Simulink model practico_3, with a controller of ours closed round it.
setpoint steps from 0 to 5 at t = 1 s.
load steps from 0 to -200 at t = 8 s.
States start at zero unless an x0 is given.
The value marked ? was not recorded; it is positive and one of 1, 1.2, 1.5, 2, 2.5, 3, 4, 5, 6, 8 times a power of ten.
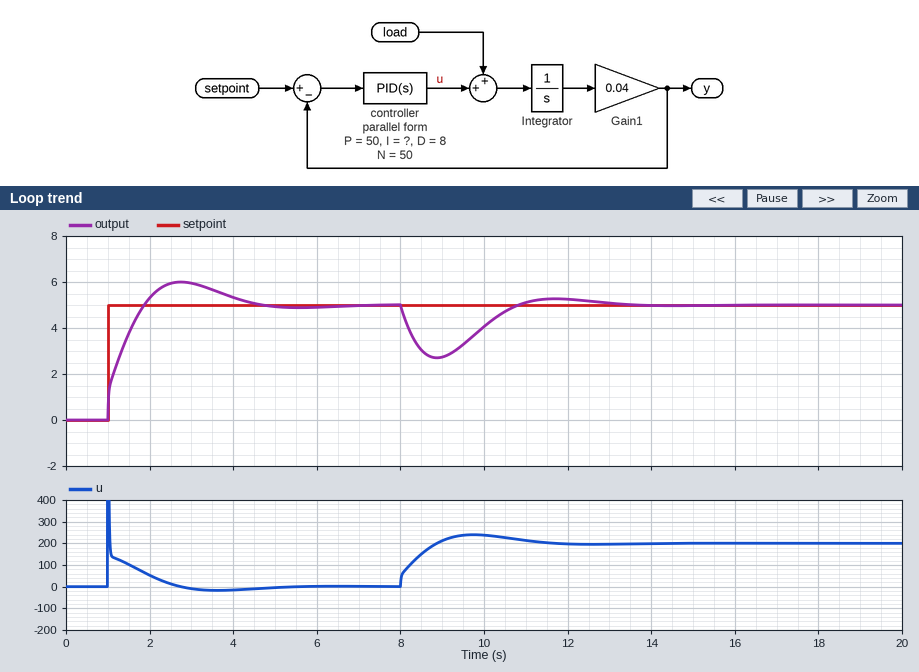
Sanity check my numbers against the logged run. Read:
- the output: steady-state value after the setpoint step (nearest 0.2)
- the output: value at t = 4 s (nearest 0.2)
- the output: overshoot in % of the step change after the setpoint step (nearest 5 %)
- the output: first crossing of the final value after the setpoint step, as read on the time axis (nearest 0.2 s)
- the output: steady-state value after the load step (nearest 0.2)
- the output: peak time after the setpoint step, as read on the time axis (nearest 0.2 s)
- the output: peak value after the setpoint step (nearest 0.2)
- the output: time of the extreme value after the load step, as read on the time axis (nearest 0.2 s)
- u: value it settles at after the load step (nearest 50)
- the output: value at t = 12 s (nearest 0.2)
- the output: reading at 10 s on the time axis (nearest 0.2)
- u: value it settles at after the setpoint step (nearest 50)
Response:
5.0
5.4
20 %
1.8 s
5.0
2.8 s
6.0
8.8 s
200
5.2
4.0
0
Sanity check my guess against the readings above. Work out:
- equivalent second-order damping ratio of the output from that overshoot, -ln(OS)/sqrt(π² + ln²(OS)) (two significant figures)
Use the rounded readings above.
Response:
0.46
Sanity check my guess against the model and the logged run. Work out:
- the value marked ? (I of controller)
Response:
60
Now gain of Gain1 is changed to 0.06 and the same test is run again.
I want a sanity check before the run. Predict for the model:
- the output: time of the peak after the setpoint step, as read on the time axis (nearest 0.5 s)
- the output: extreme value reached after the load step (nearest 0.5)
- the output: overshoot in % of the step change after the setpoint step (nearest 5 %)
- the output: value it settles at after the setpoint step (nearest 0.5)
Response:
2.5 s
2.5
15 %
5.0
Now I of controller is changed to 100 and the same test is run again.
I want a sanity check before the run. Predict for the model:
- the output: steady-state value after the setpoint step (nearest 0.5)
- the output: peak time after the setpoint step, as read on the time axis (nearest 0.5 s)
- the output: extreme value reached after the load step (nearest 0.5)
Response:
5.0
2.5 s
3.0
